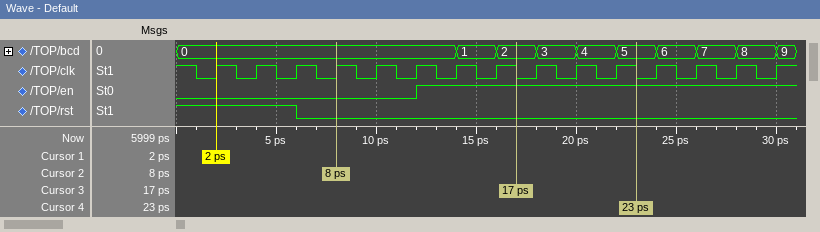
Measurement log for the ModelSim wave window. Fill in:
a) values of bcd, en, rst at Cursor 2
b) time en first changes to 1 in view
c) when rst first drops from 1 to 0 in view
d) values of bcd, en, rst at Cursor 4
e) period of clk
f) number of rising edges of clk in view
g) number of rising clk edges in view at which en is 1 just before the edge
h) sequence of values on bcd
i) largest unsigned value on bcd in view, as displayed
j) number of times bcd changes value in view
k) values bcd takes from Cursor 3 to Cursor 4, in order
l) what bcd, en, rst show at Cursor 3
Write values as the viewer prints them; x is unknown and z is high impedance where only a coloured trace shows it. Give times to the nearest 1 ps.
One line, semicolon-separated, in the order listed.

bcd=0, en=0, rst=0; 12 ps; 6 ps; bcd=5, en=1, rst=0; 2 ps; 15; 9; 0, 1, 2, 3, 4, 5, 6, 7, 8, 9; 9; 9; 2, 3, 4, 5; bcd=2, en=1, rst=0
